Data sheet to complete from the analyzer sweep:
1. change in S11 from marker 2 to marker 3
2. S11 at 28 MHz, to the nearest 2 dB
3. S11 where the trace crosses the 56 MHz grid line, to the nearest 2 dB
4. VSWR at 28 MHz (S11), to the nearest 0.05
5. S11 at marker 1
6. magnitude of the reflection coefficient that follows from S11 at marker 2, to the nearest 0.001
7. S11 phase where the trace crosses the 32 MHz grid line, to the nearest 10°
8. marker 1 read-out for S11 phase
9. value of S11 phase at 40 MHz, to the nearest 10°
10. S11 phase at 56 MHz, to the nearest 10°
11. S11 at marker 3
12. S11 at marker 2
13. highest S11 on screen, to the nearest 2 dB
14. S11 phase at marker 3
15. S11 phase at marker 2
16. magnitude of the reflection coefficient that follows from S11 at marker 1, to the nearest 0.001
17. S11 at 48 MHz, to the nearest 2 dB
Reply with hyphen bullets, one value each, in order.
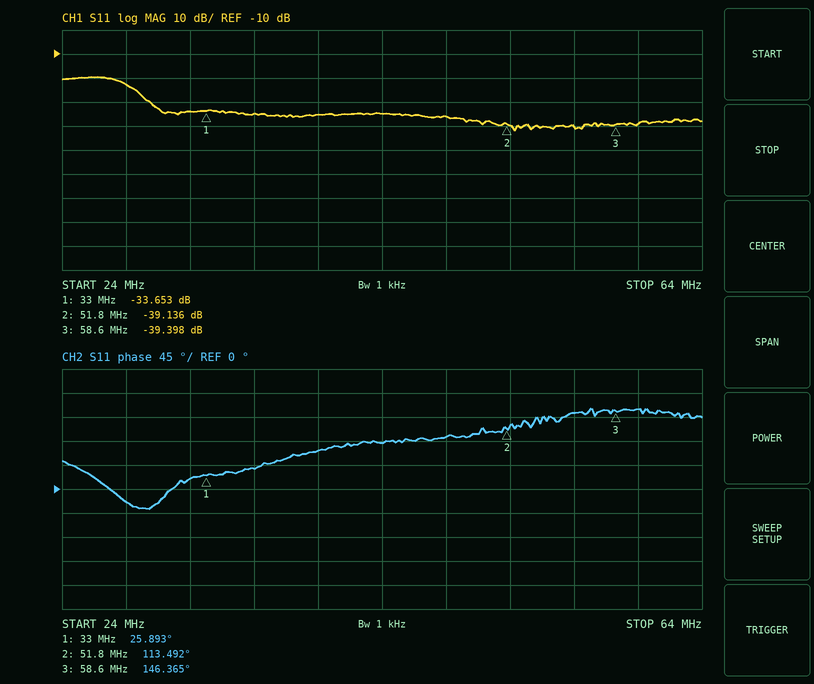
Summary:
- -0.262 dB
- -22 dB
- -40 dB
- 1.15
- -33.653 dB
- 0.011
- 20°
- 25.893°
- 70°
- 140°
- -39.398 dB
- -39.136 dB
- -20 dB
- 146.365°
- 113.492°
- 0.021
- -36 dB
